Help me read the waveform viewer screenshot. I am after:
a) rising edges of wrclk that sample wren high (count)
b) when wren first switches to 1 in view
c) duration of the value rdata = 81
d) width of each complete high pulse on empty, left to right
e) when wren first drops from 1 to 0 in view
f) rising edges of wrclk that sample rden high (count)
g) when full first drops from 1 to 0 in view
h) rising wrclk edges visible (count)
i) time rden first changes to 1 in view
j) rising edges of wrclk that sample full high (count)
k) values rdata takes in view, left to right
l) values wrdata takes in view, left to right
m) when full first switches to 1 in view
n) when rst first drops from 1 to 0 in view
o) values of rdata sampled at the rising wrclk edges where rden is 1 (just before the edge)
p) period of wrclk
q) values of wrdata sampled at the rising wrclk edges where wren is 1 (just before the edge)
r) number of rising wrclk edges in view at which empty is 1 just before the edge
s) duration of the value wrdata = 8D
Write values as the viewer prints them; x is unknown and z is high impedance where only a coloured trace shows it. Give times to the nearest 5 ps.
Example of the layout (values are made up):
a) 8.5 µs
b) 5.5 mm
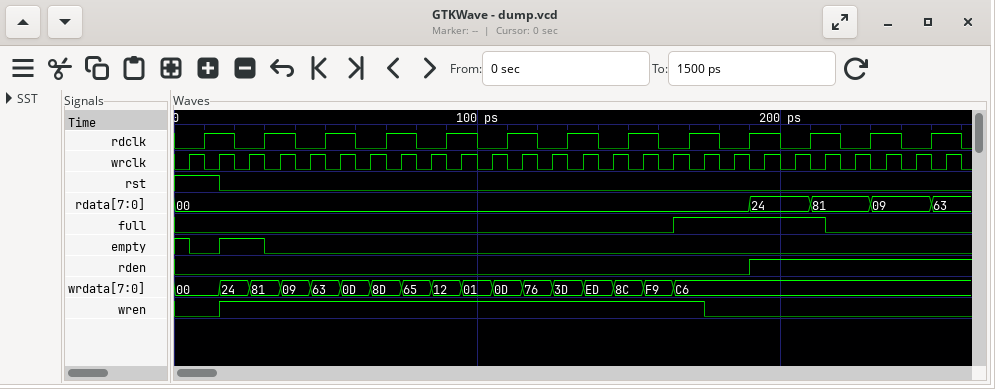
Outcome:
a) 16
b) 15 ps
c) 20 ps
d) 15 ps
e) 175 ps
f) 7
g) 215 ps
h) 26
i) 190 ps
j) 5
k) 00, 24, 81, 09, 63
l) 00, 24, 81, 09, 63, 0D, 8D, 65, 12, 01, 0D, 76, 3D, ED, 8C, F9, C6
m) 165 ps
n) 15 ps
o) 24, 24, 81, 81, 09, 09, 63
p) 10 ps
q) 24, 81, 09, 63, 0D, 8D, 65, 12, 01, 0D, 76, 3D, ED, 8C, F9, C6
r) 2
s) 10 ps
